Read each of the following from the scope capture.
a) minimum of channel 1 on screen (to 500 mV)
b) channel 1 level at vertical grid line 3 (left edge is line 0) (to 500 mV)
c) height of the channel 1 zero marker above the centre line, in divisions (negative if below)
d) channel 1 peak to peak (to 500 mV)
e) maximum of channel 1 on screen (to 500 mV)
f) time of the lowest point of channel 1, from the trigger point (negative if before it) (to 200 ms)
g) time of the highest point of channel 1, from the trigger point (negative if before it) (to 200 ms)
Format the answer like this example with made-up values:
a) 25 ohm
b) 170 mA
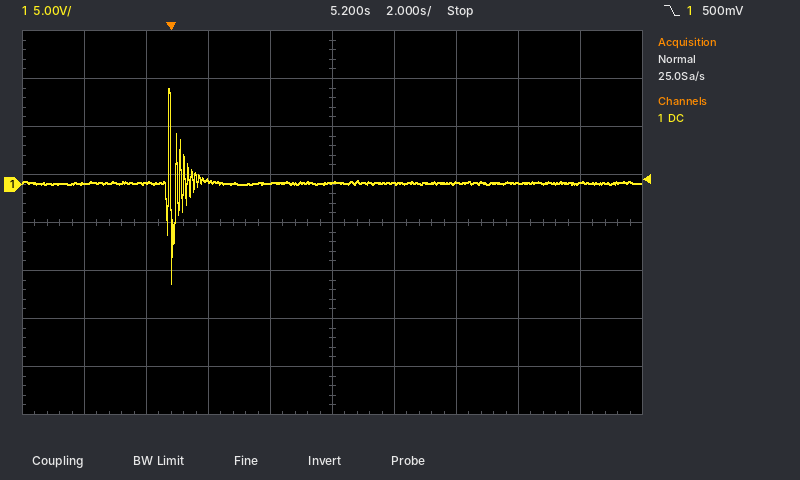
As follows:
a) -10.5 V
b) 500 mV
c) +0.8 div
d) 20.5 V
e) 10.0 V
f) 0.0 s
g) 0.0 s
